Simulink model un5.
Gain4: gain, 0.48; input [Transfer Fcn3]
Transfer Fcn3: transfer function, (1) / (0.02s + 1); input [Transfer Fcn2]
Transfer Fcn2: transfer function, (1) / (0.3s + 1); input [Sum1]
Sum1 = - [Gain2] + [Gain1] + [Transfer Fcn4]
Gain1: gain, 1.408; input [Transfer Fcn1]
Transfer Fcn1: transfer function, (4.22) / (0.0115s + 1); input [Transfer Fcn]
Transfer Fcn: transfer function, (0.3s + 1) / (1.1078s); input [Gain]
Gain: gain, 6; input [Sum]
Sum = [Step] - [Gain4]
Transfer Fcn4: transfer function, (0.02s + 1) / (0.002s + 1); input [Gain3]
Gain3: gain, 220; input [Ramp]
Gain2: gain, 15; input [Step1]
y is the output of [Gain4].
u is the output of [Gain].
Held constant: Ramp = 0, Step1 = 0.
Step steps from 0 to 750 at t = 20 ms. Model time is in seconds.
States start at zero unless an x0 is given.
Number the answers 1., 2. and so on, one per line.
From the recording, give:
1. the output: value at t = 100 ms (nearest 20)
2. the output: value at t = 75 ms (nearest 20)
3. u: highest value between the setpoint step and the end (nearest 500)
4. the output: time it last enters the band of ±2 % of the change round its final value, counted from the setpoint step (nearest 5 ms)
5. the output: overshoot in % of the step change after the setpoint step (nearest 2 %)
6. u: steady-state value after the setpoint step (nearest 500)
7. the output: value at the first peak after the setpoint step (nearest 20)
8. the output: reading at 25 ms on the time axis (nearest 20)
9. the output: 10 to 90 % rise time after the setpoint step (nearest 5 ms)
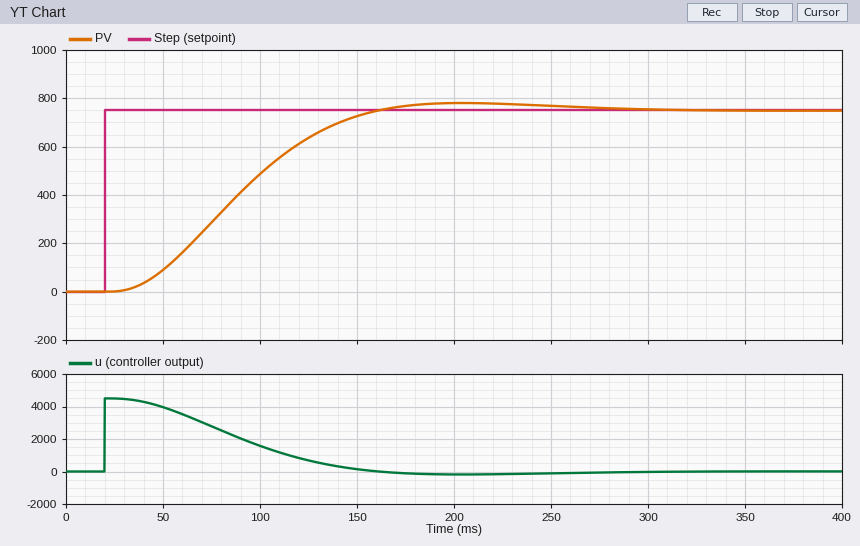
1. 480
2. 280
3. 4500
4. 240 ms
5. 4 %
6. 0
7. 780
8. 0
9. 85 ms
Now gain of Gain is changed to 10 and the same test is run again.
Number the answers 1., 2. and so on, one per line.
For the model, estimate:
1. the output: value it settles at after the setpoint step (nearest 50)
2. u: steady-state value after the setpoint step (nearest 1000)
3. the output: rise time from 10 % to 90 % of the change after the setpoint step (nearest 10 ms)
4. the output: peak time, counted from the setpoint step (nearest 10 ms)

1. 750
2. 0
3. 50 ms
4. 120 ms
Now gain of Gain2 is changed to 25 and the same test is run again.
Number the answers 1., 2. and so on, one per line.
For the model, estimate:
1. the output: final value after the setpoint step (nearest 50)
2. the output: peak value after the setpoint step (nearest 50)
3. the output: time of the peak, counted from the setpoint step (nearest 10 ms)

1. 750
2. 800
3. 180 ms
